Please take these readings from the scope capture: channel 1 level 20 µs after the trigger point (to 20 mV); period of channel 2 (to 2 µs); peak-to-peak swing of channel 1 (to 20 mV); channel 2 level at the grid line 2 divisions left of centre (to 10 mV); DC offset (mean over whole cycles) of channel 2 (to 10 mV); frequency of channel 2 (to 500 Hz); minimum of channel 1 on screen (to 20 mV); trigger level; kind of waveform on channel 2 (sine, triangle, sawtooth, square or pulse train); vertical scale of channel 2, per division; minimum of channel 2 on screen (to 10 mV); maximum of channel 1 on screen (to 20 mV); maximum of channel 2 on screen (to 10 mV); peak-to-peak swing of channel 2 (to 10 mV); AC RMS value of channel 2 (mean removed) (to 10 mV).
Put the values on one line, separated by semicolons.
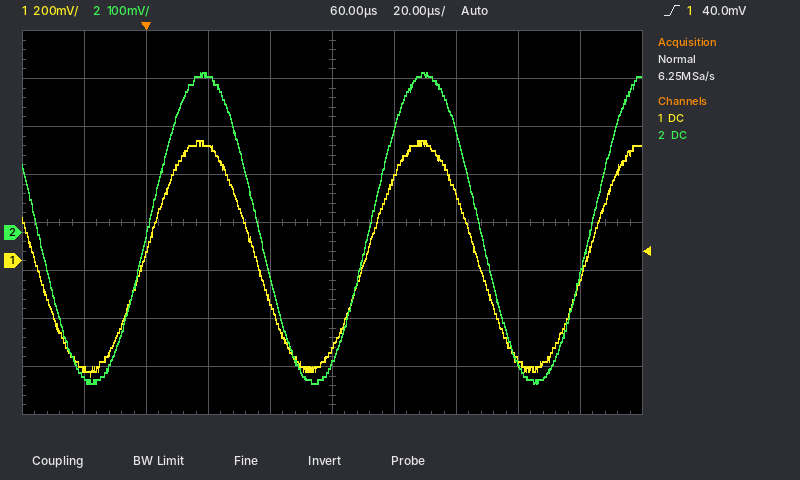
480 mV; 72 µs; 980 mV; 330 mV; 10 mV; 14.0 kHz; -480 mV; 40.0 mV; sine; 100 mV; -320 mV; 500 mV; 330 mV; 650 mV; 230 mV
